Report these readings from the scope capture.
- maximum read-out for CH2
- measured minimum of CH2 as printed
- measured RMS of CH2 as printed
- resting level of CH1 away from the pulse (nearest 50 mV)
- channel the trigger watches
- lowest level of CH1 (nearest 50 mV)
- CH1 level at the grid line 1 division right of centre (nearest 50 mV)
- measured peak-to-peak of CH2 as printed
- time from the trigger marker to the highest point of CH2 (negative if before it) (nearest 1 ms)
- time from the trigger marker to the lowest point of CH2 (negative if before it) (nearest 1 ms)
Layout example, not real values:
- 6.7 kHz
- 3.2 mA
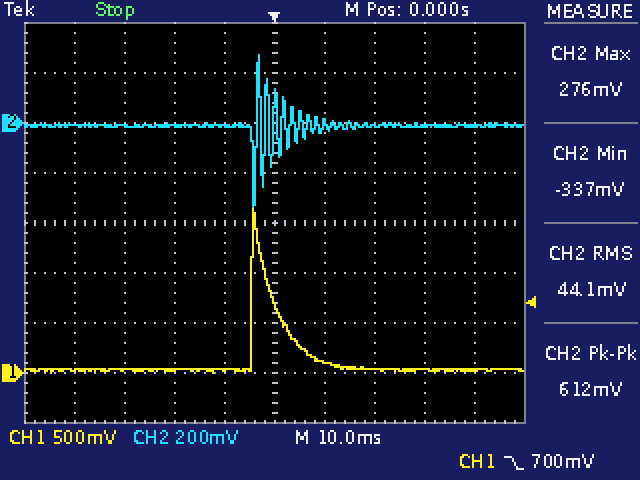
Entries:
- 276 mV
- -337 mV
- 44.1 mV
- 50 mV
- CH1
- 0 mV
- 100 mV
- 612 mV
- -3 ms
- -4 ms
